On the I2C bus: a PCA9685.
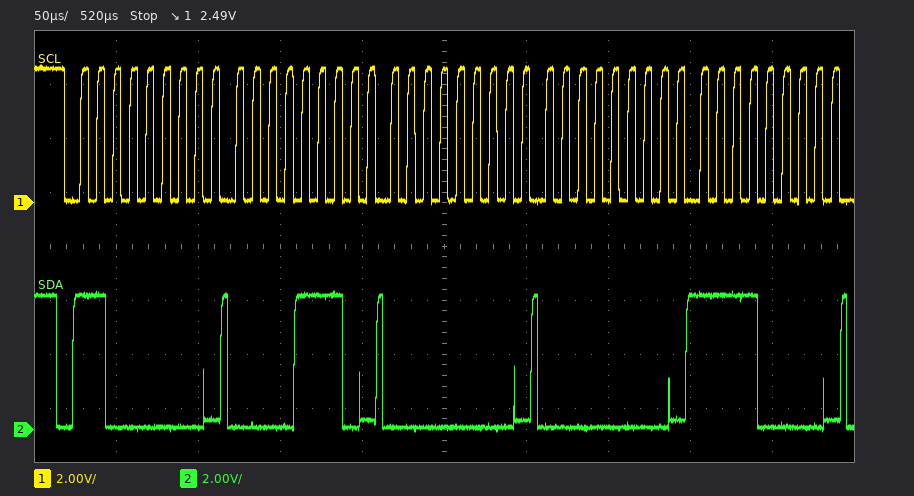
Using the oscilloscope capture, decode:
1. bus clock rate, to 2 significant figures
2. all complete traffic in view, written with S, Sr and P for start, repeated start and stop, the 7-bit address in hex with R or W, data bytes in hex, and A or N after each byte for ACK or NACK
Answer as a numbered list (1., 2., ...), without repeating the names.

1. 100 kHz
2. S 60W A 0E A 00 A 00 A F0 A
